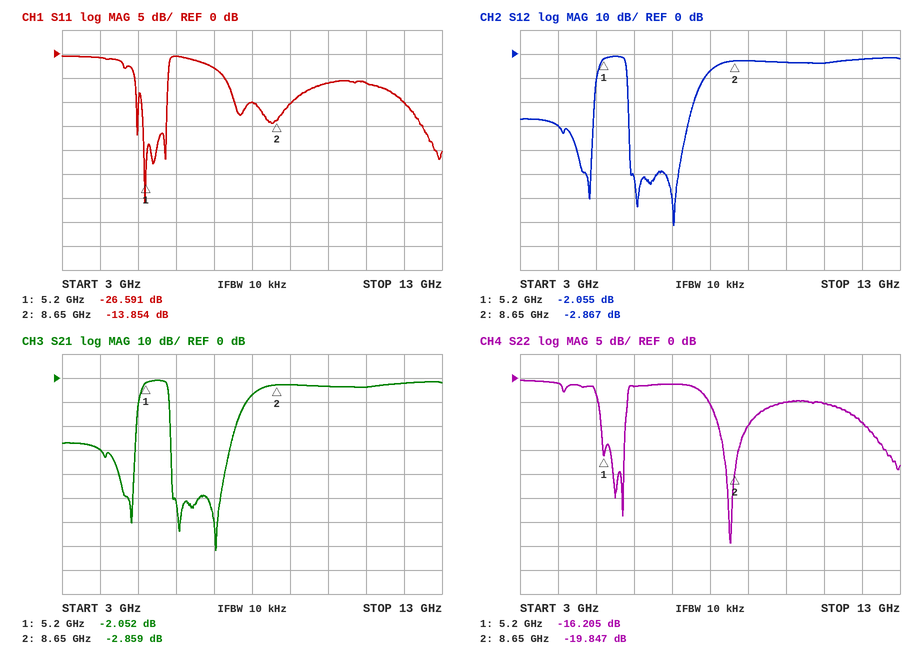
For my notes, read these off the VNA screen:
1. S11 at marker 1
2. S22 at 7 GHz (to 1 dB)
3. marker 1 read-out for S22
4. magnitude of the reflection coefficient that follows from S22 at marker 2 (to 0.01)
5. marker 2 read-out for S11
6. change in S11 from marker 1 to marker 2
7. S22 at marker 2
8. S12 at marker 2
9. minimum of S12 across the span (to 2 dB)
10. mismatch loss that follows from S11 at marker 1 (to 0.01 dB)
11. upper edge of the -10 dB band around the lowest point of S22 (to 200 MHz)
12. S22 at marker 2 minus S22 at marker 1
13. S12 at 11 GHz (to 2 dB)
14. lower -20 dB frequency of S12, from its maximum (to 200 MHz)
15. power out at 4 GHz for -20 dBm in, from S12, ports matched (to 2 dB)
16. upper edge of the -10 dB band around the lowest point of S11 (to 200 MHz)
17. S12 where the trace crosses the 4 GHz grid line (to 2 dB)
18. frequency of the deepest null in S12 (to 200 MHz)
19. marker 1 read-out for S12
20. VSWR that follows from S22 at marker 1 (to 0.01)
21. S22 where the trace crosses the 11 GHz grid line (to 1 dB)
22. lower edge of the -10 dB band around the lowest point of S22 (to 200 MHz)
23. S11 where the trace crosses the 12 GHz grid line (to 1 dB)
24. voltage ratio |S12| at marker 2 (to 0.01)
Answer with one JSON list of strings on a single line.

["-26.591 dB", "-1 dB", "-16.205 dB", "0.10", "-13.854 dB", "12.737 dB", "-19.847 dB", "-2.867 dB", "-72 dB", "0.01 dB", "9.0 GHz", "-3.642 dB", "-4 dB", "5.0 GHz", "-50 dBm", "5.8 GHz", "-30 dB", "7.0 GHz", "-2.055 dB", "1.37", "-5 dB", "8.2 GHz", "-10 dB", "0.72"]
